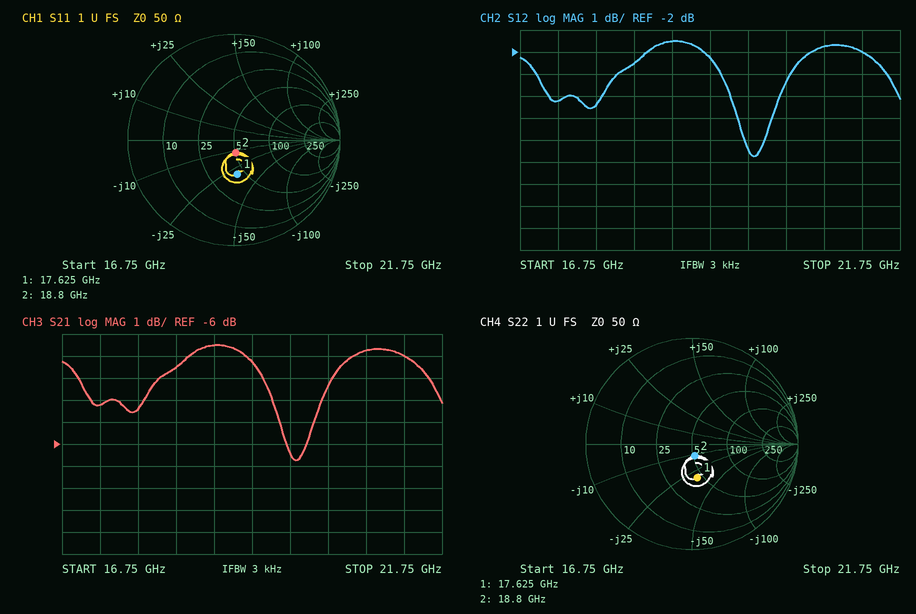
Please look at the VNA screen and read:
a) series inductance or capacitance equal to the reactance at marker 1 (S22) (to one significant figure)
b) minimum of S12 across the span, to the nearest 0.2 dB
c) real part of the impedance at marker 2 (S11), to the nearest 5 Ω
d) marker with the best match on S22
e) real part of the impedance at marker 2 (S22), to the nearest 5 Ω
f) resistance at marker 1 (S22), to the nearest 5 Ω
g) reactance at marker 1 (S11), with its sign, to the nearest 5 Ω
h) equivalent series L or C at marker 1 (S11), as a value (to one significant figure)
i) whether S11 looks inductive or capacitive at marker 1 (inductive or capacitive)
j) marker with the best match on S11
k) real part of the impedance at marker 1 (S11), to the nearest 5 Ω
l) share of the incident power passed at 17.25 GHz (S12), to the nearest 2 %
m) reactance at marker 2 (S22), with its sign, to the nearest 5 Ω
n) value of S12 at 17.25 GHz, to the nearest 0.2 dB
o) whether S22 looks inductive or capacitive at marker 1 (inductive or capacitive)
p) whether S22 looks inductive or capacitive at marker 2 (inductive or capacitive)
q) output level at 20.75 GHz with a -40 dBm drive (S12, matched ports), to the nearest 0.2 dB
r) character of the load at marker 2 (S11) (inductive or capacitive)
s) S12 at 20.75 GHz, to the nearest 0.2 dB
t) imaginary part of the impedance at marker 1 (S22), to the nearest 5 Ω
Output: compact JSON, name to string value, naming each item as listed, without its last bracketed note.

{"series inductance or capacitance equal to the reactance at marker 1 (S22)": "300 fF", "minimum of S12 across the span, to the nearest 0.2 dB": "-6.8 dB", "real part of the impedance at marker 2 (S11), to the nearest 5 Ω": "50 Ω", "marker with the best match on S22": "marker 2", "real part of the impedance at marker 2 (S22), to the nearest 5 Ω": "50 Ω", "resistance at marker 1 (S22), to the nearest 5 Ω": "45 Ω", "reactance at marker 1 (S11), with its sign, to the nearest 5 Ω": "-30 Ω", "equivalent series L or C at marker 1 (S11), as a value": "300 fF", "whether S11 looks inductive or capacitive at marker 1": "capacitive", "marker with the best match on S11": "marker 2", "real part of the impedance at marker 1 (S11), to the nearest 5 Ω": "45 Ω", "share of the incident power passed at 17.25 GHz (S12), to the nearest 2 %": "38 %", "reactance at marker 2 (S22), with its sign, to the nearest 5 Ω": "-10 Ω", "value of S12 at 17.25 GHz, to the nearest 0.2 dB": "-4.2 dB", "whether S22 looks inductive or capacitive at marker 1": "capacitive", "whether S22 looks inductive or capacitive at marker 2": "capacitive", "output level at 20.75 GHz with a -40 dBm drive (S12, matched ports), to the nearest 0.2 dB": "-41.8 dBm", "character of the load at marker 2 (S11)": "capacitive", "S12 at 20.75 GHz, to the nearest 0.2 dB": "-1.8 dB", "imaginary part of the impedance at marker 1 (S22), to the nearest 5 Ω": "-30 Ω"}
